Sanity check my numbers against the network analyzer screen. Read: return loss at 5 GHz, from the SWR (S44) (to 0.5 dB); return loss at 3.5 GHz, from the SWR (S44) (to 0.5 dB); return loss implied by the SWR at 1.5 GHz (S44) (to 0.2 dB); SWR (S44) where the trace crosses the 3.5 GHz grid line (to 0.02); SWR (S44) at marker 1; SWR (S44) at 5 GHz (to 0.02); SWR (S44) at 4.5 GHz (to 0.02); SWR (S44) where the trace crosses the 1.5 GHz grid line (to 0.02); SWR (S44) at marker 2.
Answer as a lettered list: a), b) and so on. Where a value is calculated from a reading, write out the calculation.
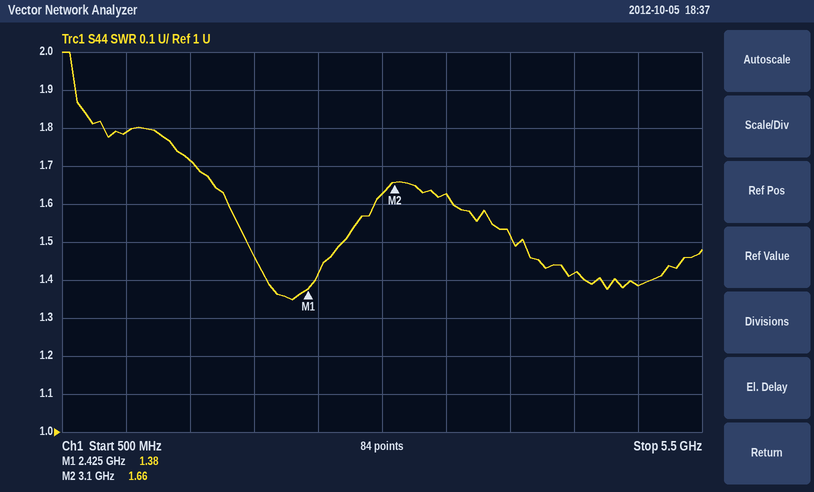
a) −20 log10((1.38 − 1)/(1.38 + 1)) ≈ 15.9 dB, so 16.0 dB to the nearest 0.5 dB
b) −20 log10((1.62 − 1)/(1.62 + 1)) ≈ 12.5 dB
c) −20 log10((1.72 − 1)/(1.72 + 1)) ≈ 11.5 dB, so 11.6 dB to the nearest 0.2 dB
d) 1.62
e) 1.38
f) 1.38
g) 1.42
h) 1.72
i) 1.66
